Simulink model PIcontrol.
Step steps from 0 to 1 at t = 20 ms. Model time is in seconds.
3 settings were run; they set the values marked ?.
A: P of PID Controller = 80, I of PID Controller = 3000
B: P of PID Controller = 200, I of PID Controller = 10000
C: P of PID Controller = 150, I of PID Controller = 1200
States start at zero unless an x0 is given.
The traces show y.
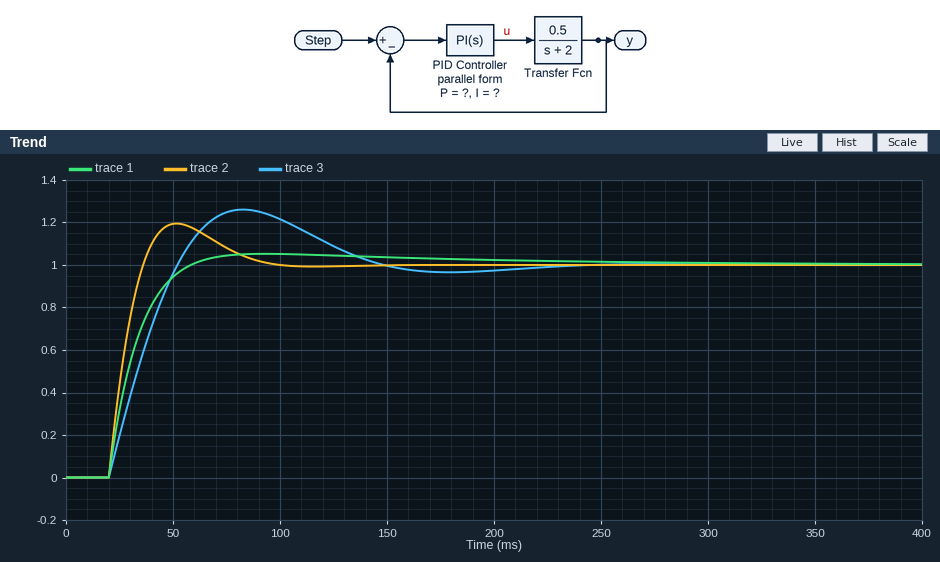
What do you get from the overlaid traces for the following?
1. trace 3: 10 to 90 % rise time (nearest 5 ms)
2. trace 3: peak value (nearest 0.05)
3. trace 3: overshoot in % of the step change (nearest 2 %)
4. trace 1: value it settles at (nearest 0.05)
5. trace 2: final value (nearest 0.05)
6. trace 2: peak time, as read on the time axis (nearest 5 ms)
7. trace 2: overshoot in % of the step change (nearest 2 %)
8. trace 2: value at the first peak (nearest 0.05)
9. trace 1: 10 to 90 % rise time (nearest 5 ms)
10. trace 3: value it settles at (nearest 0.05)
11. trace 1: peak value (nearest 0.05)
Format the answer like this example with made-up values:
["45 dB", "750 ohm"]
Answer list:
["25 ms", "1.25", "26 %", "1.00", "1.00", "50 ms", "20 %", "1.20", "25 ms", "1.00", "1.05"]
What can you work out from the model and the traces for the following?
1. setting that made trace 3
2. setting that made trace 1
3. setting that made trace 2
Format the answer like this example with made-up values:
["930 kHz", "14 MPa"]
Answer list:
["A", "C", "B"]
